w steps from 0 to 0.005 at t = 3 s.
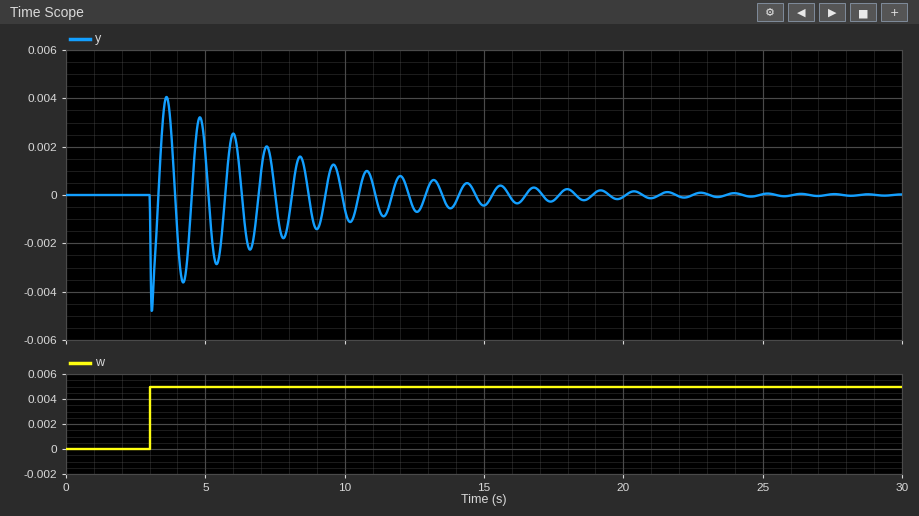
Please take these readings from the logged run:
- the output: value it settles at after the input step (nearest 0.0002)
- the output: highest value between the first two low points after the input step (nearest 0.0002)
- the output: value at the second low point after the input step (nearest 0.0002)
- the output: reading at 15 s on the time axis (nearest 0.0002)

0.0000
0.0040
-0.0036
-0.0004
